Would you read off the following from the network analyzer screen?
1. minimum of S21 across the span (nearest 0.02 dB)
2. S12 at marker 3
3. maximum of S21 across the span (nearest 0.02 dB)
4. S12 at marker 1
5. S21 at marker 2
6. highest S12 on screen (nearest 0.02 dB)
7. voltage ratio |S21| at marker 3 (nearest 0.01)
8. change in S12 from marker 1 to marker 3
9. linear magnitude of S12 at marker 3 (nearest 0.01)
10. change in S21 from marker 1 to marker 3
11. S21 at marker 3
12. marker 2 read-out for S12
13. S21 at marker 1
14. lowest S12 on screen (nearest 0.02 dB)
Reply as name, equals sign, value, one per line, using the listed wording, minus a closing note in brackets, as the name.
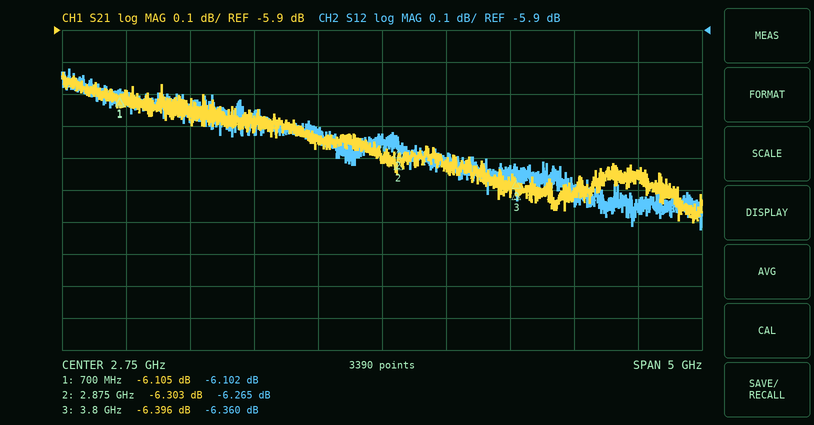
minimum of S21 across the span = -6.50 dB
S12 at marker 3 = -6.360 dB
maximum of S21 across the span = -6.04 dB
S12 at marker 1 = -6.102 dB
S21 at marker 2 = -6.303 dB
highest S12 on screen = -6.02 dB
voltage ratio |S21| at marker 3 = 0.48
change in S12 from marker 1 to marker 3 = -0.258 dB
linear magnitude of S12 at marker 3 = 0.48
change in S21 from marker 1 to marker 3 = -0.291 dB
S21 at marker 3 = -6.396 dB
marker 2 read-out for S12 = -6.265 dB
S21 at marker 1 = -6.105 dB
lowest S12 on screen = -6.52 dB
